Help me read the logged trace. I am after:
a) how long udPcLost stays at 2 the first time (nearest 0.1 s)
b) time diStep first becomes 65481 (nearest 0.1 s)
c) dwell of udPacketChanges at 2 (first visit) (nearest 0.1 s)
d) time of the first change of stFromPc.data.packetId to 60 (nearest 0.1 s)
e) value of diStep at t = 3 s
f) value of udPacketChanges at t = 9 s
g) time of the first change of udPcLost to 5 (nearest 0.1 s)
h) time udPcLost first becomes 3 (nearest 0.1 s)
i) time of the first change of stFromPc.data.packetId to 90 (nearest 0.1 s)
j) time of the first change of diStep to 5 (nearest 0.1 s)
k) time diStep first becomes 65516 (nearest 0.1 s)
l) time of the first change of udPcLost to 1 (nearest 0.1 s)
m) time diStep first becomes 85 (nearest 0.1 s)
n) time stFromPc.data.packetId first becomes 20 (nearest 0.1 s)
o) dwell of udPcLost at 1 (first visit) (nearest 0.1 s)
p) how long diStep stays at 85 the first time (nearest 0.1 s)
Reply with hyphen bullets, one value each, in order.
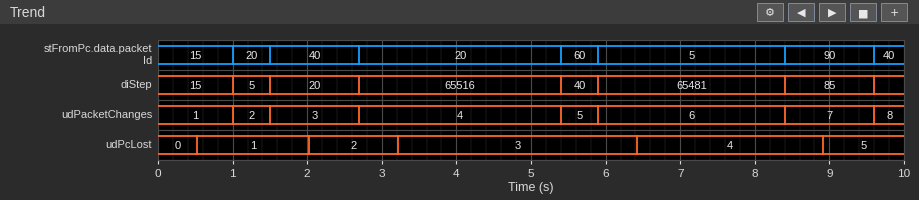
- 1.2 s
- 5.9 s
- 0.5 s
- 5.4 s
- 65516
- 7
- 8.9 s
- 3.2 s
- 8.4 s
- 1.0 s
- 2.7 s
- 0.5 s
- 8.4 s
- 1.0 s
- 1.5 s
- 1.2 s
